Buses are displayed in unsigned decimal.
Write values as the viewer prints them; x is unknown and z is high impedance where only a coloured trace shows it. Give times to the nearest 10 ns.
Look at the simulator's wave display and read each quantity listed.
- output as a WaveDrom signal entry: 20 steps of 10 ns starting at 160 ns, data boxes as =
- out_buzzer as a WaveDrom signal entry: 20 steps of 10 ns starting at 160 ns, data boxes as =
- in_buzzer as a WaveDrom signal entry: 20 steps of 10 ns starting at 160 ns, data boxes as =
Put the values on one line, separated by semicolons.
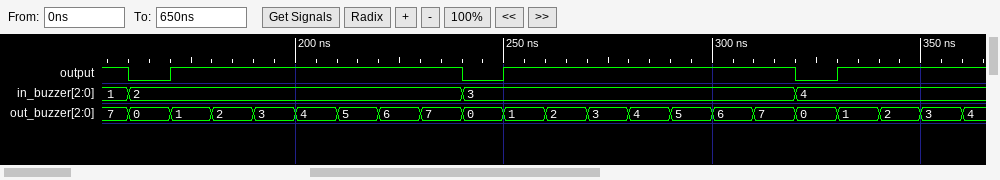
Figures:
{name: 'output', wave: '01......01......01..'}; {name: 'out_buzzer', wave: '====================', data: '0 1 2 3 4 5 6 7 0 1 2 3 4 5 6 7 0 1 2 3'}; {name: 'in_buzzer', wave: '=.......=.......=...', data: '2 3 4'}
